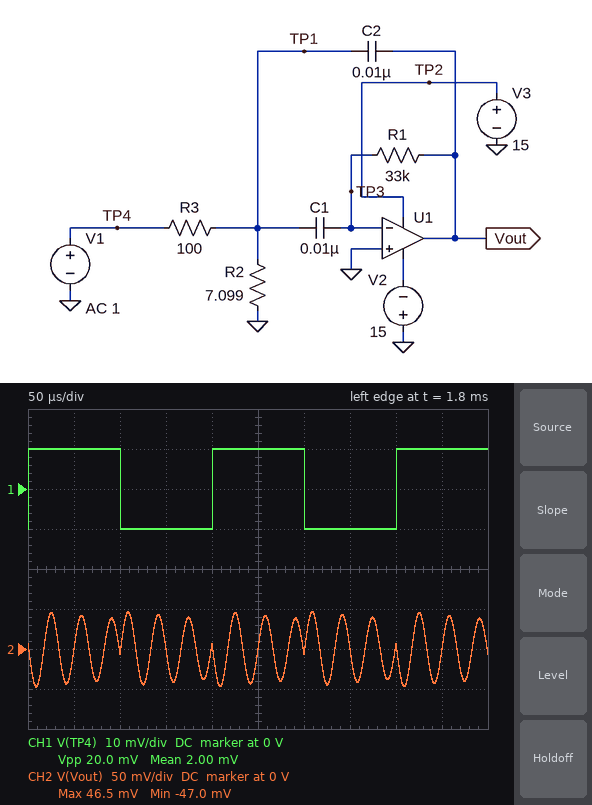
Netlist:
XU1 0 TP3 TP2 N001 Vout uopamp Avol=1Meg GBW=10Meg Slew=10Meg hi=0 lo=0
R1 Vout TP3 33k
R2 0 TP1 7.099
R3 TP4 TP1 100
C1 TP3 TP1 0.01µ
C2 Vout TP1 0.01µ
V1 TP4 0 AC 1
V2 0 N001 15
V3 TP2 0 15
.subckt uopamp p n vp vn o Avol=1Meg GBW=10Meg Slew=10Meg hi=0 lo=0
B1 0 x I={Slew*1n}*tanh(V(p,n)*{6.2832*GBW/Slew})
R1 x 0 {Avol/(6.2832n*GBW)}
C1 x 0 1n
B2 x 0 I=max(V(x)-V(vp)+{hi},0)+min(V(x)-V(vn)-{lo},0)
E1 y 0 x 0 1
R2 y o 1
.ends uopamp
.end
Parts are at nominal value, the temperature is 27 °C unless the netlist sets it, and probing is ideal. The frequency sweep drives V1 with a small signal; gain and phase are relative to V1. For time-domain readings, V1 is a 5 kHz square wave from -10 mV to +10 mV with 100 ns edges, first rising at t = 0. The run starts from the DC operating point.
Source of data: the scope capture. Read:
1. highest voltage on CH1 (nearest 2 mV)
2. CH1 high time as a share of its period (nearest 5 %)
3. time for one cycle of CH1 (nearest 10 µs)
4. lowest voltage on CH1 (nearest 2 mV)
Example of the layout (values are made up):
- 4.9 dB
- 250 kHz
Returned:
- 10 mV
- 50 %
- 200 µs
- -10 mV
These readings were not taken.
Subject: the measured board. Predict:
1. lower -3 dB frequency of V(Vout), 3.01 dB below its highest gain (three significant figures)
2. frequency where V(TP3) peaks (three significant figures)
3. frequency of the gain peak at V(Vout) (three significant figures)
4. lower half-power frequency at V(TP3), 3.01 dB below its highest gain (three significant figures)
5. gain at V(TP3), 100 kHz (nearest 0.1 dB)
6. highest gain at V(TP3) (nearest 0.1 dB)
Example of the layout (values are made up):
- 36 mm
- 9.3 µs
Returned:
- 30.2 kHz
- 30.6 kHz
- 30.6 kHz
- 30.2 kHz
- -37.0 dB
- -6.0 dB
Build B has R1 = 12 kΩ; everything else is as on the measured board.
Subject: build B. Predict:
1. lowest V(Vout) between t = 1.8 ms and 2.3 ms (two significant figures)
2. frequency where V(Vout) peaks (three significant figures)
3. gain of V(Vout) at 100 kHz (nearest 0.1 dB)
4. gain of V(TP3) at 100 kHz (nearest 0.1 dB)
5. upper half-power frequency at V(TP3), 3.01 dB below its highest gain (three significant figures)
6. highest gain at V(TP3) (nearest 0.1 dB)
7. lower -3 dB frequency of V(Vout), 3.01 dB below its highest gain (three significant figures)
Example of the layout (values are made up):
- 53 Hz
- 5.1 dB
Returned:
- -33 mV
- 50.7 kHz
- 4.7 dB
- -35.3 dB
- 51.8 kHz
- -10.4 dB
- 49.6 kHz
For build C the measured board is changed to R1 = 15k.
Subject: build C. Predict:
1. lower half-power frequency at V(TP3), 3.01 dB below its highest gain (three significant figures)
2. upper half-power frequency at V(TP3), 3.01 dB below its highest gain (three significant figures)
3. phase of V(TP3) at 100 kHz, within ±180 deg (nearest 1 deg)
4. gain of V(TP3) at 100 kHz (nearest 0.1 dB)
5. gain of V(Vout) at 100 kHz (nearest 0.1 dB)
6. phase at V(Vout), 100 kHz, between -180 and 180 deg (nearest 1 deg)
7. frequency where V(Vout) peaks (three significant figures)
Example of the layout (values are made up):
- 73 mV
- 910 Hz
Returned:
- 44.5 kHz
- 46.2 kHz
- 1 deg
- -35.8 dB
- 4.2 dB
- 91 deg
- 45.3 kHz
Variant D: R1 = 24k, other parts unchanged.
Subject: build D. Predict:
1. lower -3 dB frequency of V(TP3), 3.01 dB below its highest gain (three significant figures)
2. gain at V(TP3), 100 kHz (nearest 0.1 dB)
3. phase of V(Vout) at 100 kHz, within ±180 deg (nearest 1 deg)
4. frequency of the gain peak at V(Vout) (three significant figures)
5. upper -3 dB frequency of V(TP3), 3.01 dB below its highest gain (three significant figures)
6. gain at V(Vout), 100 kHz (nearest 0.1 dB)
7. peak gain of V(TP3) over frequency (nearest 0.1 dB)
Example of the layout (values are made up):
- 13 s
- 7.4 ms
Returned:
- 35.3 kHz
- -36.6 dB
- 90 deg
- 35.8 kHz
- 36.4 kHz
- 3.4 dB
- -7.4 dB
